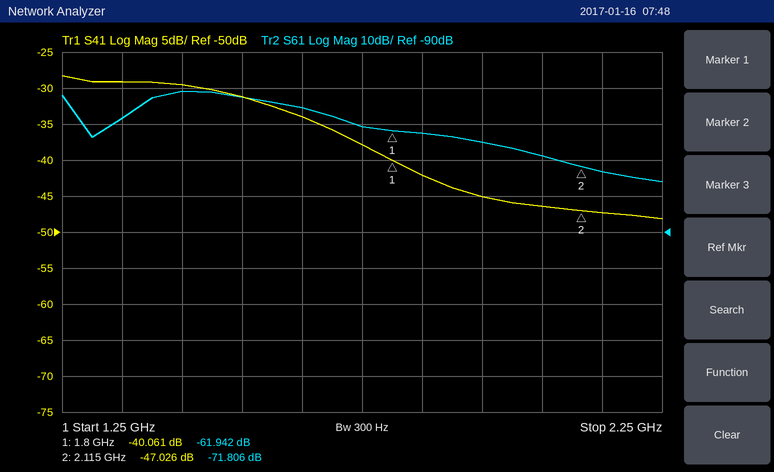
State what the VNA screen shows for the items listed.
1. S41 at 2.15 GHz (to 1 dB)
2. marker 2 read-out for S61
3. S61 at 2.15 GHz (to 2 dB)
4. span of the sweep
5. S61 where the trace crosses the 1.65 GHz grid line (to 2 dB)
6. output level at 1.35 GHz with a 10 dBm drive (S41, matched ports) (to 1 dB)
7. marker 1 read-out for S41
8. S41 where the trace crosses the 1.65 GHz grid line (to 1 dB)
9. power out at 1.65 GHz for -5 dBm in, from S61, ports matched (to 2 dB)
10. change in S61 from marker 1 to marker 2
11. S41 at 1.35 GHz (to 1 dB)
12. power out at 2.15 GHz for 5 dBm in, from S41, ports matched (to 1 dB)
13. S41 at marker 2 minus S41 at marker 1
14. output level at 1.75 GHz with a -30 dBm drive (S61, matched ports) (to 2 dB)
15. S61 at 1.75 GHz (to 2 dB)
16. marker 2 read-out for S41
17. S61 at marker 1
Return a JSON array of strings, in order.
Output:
["-47 dB", "-71.806 dB", "-74 dB", "1 GHz", "-56 dB", "-19 dBm", "-40.061 dB", "-34 dB", "-60 dBm", "-9.864 dB", "-29 dB", "-42 dBm", "-6.965 dB", "-90 dBm", "-60 dB", "-47.026 dB", "-61.942 dB"]
